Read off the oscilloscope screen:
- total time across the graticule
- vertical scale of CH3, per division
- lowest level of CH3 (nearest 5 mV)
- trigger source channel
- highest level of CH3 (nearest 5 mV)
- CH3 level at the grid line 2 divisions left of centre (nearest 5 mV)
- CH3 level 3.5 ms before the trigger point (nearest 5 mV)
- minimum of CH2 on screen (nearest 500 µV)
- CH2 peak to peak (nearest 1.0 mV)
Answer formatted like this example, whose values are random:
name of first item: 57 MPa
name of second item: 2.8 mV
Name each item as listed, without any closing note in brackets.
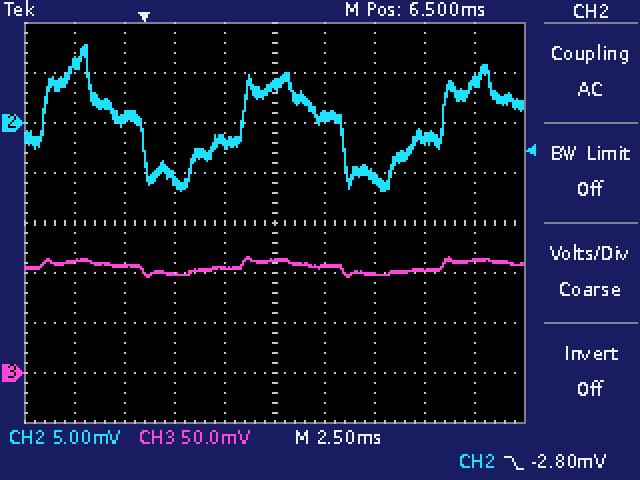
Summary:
total time across the graticule: 25 ms
vertical scale of CH3, per division: 50 mV
lowest level of CH3: 95 mV
trigger source channel: CH2
highest level of CH3: 115 mV
CH3 level at the grid line 2 divisions left of centre: 100 mV
CH3 level 3.5 ms before the trigger point: 110 mV
minimum of CH2 on screen: -7.0 mV
CH2 peak to peak: 15.0 mV
